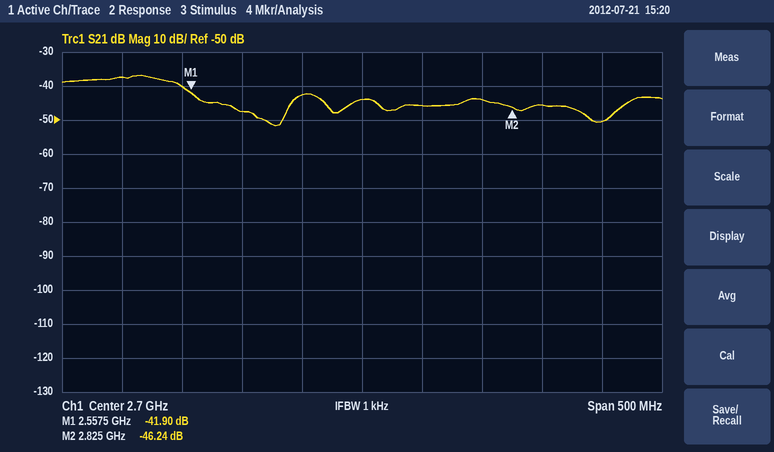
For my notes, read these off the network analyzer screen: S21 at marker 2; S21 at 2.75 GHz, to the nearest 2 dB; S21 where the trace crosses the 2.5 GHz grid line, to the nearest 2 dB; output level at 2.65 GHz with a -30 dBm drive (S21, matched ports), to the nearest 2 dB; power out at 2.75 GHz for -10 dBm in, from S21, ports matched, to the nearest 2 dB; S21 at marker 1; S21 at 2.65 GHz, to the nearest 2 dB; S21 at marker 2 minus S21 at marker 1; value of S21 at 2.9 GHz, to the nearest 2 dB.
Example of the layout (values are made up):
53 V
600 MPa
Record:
-46.24 dB
-46 dB
-38 dB
-72 dBm
-56 dBm
-41.90 dB
-42 dB
-4.34 dB
-50 dB
